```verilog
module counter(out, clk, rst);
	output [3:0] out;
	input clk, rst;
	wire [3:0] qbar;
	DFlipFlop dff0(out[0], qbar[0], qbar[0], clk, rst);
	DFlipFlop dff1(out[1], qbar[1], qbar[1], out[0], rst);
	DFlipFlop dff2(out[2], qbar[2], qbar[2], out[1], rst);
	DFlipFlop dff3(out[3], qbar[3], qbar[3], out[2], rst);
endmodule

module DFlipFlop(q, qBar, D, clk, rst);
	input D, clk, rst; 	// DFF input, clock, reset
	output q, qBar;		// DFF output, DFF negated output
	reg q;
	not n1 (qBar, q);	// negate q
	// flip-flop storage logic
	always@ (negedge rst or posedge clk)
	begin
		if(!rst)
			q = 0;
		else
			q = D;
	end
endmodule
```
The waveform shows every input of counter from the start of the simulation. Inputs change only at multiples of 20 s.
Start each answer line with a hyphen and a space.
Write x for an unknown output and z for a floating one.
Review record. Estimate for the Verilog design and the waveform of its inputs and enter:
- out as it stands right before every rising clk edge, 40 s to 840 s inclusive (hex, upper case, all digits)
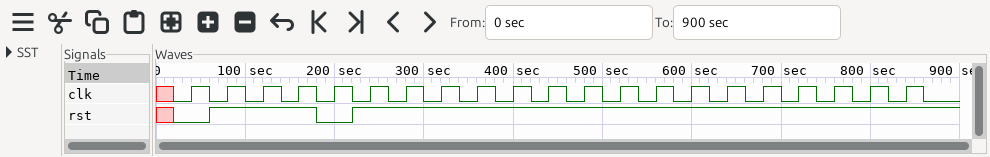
- 0, 0, F, E, 0, 0, F, E, D, C, B, A, 9, 8, 7, 6, 5, 4, 3, 2, 1
